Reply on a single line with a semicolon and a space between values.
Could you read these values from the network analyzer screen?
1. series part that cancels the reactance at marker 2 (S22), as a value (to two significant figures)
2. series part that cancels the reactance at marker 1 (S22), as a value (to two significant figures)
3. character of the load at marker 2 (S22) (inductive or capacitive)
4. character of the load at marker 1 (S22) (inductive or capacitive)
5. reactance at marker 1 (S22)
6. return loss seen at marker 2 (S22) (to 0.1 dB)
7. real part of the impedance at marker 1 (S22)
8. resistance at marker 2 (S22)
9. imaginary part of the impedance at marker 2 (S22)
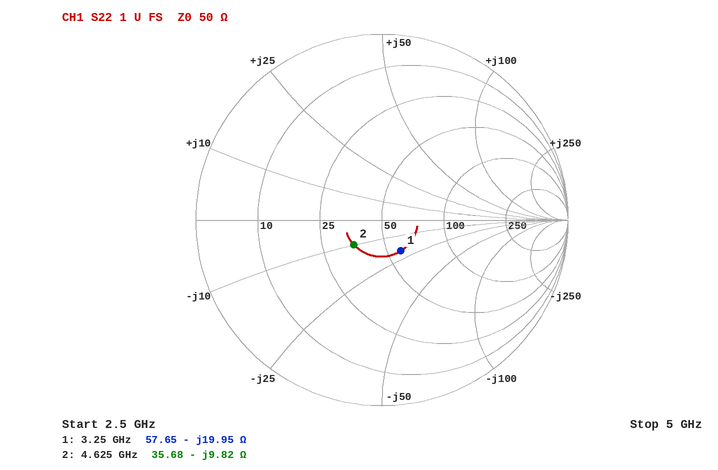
340 pH; 980 pH; capacitive; capacitive; -19.95 Ω; 13.9 dB; 57.65 Ω; 35.68 Ω; -9.82 Ω
